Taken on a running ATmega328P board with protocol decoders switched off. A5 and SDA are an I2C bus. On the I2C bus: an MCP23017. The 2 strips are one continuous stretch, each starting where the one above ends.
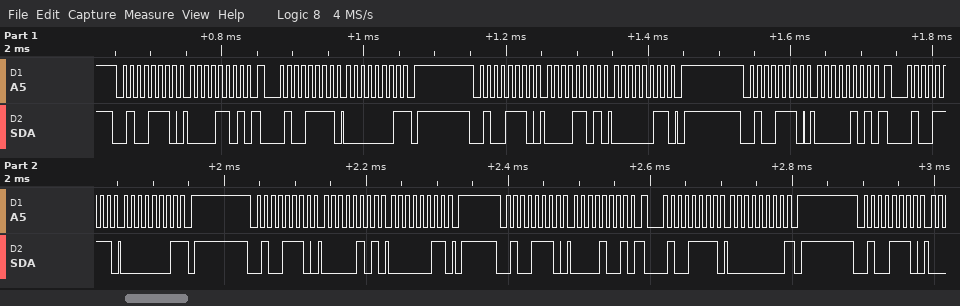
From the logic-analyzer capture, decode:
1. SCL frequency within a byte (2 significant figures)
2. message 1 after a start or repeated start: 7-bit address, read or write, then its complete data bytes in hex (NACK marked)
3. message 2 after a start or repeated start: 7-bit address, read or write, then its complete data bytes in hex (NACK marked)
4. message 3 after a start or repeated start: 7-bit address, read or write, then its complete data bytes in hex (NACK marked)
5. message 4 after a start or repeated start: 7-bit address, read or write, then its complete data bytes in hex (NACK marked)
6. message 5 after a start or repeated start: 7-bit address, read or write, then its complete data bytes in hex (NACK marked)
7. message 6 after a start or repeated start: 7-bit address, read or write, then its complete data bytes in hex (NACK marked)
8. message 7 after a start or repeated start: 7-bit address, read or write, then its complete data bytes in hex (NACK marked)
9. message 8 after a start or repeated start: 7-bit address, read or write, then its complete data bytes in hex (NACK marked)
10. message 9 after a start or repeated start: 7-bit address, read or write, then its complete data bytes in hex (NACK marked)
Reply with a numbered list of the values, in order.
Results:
1. 100 kHz
2. 0x27 write: 0D
3. 0x27 read: 01 NACK
4. 0x27 write: 0D 03
5. 0x27 write: 05
6. 0x27 read: 01 NACK
7. 0x27 write: 05 03
8. 0x27 write: 09
9. 0x27 read: 00 NACK
10. 0x27 write
